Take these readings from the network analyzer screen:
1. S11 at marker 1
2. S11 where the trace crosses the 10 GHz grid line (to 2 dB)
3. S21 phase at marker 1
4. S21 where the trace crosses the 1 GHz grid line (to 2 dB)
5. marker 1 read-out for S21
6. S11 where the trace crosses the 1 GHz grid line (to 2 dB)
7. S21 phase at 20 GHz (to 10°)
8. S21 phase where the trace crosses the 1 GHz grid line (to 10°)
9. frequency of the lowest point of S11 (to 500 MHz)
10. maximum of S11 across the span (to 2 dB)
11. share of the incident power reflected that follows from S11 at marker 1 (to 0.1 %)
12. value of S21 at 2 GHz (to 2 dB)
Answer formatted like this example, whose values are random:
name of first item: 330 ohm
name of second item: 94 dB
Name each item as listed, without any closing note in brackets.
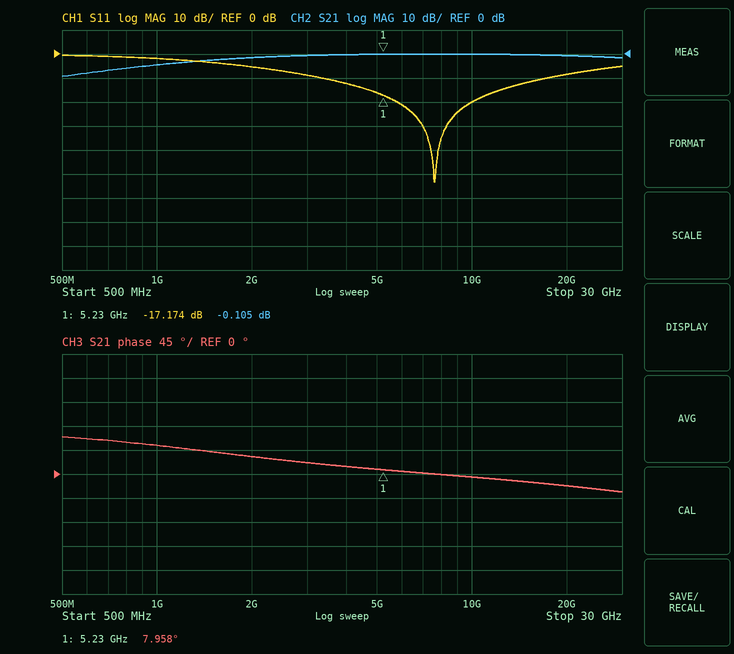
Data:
S11 at marker 1: -17.174 dB
S11 where the trace crosses the 10 GHz grid line: -20 dB
S21 phase at marker 1: 7.958°
S21 where the trace crosses the 1 GHz grid line: -4 dB
marker 1 read-out for S21: -0.105 dB
S11 where the trace crosses the 1 GHz grid line: -2 dB
S21 phase at 20 GHz: -20°
S21 phase where the trace crosses the 1 GHz grid line: 50°
frequency of the lowest point of S11: 7.5 GHz
maximum of S11 across the span: 0 dB
share of the incident power reflected that follows from S11 at marker 1: 1.9 %
value of S21 at 2 GHz: -2 dB
